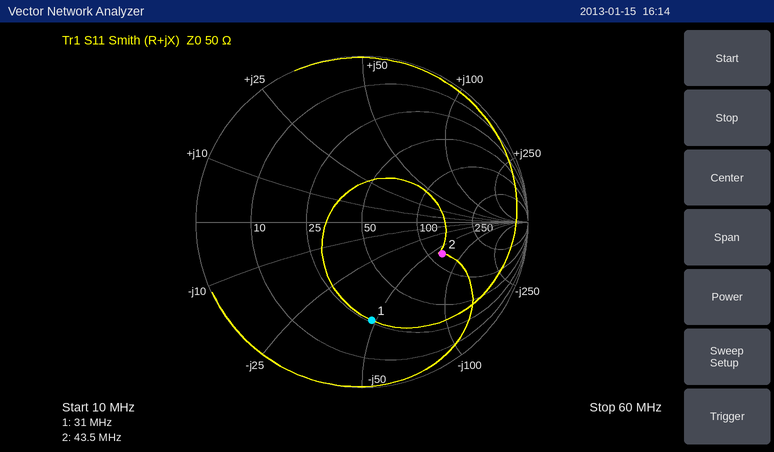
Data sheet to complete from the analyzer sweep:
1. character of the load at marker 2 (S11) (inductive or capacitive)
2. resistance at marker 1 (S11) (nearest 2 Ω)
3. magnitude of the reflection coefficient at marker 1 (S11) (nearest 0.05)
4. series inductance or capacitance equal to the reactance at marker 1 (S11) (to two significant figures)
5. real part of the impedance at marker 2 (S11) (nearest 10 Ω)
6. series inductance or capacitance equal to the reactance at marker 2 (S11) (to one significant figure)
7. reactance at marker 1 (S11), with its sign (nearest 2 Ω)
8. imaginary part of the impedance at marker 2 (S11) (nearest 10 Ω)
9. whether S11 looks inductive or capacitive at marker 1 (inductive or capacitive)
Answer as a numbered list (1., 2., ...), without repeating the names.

1. capacitive
2. 26 Ω
3. 0.60
4. 110 pF
5. 120 Ω
6. 60 pF
7. -48 Ω
8. -60 Ω
9. capacitive
